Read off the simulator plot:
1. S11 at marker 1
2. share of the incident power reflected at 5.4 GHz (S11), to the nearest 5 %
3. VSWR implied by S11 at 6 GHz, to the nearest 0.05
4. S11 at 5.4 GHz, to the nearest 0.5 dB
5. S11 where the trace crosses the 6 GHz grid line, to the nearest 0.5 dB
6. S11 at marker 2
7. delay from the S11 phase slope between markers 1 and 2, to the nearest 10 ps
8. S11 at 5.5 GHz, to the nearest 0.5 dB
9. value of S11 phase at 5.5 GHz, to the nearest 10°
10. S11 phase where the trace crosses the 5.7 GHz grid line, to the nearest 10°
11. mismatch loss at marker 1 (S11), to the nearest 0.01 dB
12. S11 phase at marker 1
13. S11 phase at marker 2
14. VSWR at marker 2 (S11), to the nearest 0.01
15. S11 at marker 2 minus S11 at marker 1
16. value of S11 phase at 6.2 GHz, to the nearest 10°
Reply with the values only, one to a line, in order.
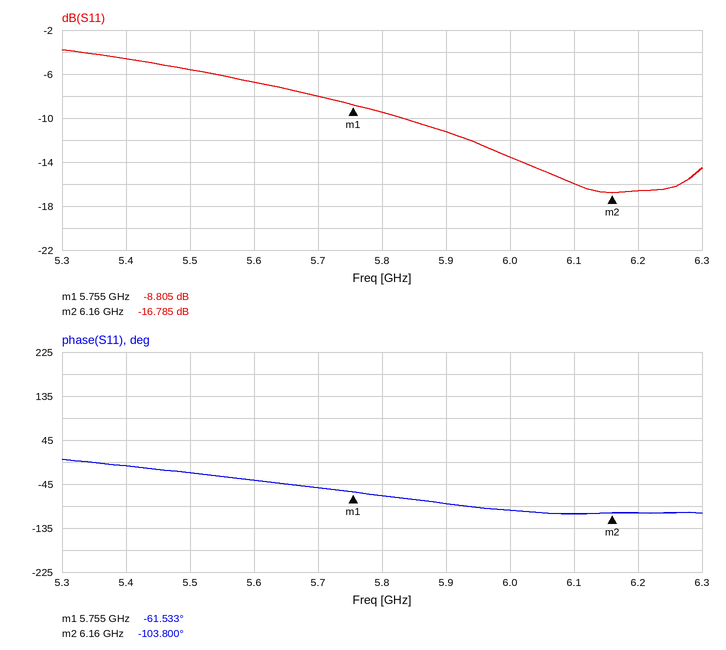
-8.805 dB
35 %
1.55
-4.5 dB
-13.5 dB
-16.785 dB
290 ps
-5.5 dB
-20°
-50°
0.61 dB
-61.533°
-103.800°
1.34
-7.980 dB
-100°
